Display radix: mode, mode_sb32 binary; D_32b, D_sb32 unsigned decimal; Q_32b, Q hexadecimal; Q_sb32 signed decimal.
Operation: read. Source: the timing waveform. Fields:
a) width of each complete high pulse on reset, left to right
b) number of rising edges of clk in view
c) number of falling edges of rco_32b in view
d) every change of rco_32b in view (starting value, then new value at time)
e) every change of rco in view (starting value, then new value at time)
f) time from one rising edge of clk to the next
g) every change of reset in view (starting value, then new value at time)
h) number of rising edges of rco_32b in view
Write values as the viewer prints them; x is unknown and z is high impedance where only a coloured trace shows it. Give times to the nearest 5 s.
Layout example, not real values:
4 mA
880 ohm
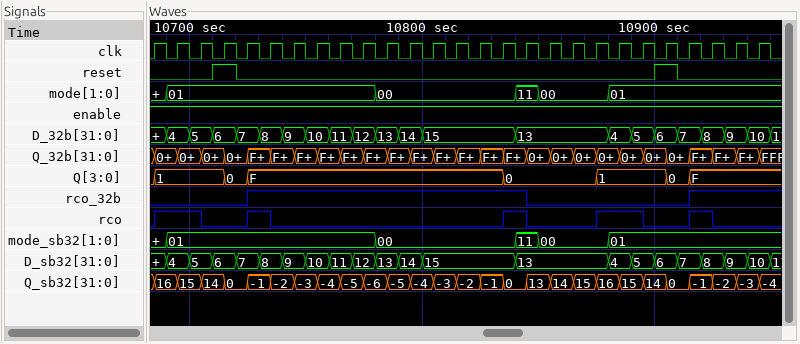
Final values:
10 s, 10 s
27
1
0, 1 at 10725 s, 0 at 10845 s, 1 at 10915 s
0, 1 at 10685 s, 0 at 10705 s, 1 at 10725 s, 0 at 10735 s, 1 at 10835 s, 0 at 10845 s, 1 at 10875 s, 0 at 10895 s, 1 at 10915 s, 0 at 10925 s
10 s
0, 1 at 10710 s, 0 at 10720 s, 1 at 10900 s, 0 at 10910 s
2
